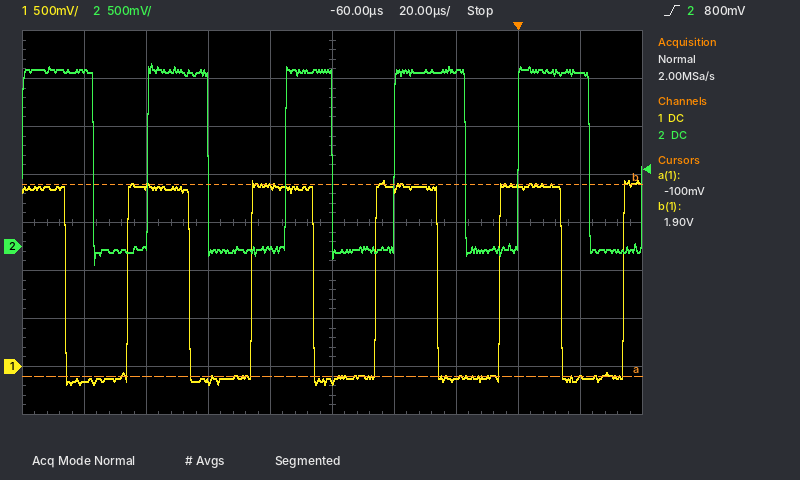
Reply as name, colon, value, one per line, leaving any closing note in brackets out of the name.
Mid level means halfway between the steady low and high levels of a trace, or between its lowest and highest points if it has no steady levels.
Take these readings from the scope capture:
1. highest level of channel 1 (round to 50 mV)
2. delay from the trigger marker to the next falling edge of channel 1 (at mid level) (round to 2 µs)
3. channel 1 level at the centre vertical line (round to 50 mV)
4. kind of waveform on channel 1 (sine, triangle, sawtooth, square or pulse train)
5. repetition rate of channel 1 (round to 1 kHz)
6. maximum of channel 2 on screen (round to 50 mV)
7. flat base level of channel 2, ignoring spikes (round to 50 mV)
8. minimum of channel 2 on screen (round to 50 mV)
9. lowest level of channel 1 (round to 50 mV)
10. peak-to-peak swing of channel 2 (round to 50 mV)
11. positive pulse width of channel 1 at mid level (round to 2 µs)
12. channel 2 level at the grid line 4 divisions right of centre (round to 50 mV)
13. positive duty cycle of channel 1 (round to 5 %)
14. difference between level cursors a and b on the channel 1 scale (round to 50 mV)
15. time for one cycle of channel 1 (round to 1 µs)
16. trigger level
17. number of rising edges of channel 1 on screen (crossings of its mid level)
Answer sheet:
highest level of channel 1: 1.95 V
delay from the trigger marker to the next falling edge of channel 1 (at mid level): 14 µs
channel 1 level at the centre vertical line: -150 mV
kind of waveform on channel 1: square
repetition rate of channel 1: 25 kHz
maximum of channel 2 on screen: 1.90 V
flat base level of channel 2, ignoring spikes: -50 mV
minimum of channel 2 on screen: -200 mV
lowest level of channel 1: -200 mV
peak-to-peak swing of channel 2: 2.10 V
positive pulse width of channel 1 at mid level: 20 µs
channel 2 level at the grid line 4 divisions right of centre: 1.80 V
positive duty cycle of channel 1: 50 %
difference between level cursors a and b on the channel 1 scale: 2.00 V
time for one cycle of channel 1: 40 µs
trigger level: 800 mV
number of rising edges of channel 1 on screen: 5
